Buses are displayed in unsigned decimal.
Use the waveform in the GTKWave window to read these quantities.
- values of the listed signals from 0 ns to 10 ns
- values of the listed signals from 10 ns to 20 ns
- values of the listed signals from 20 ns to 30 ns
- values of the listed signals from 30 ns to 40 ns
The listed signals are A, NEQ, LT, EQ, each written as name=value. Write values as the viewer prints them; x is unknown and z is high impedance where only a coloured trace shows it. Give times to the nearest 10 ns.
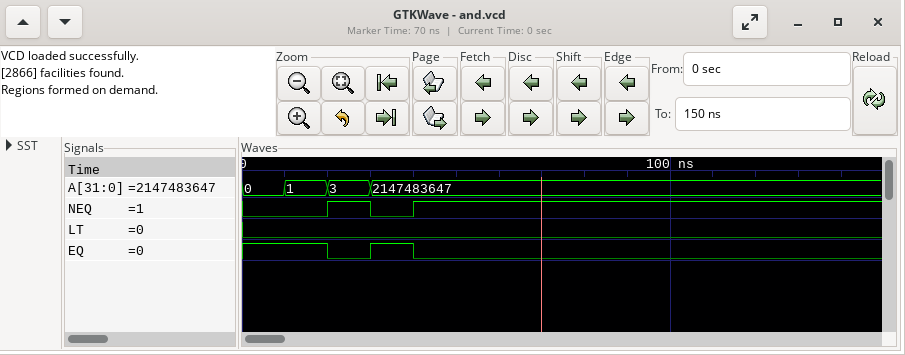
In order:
A=0, NEQ=0, LT=0, EQ=1
A=1, NEQ=0, LT=0, EQ=1
A=3, NEQ=1, LT=0, EQ=0
A=2147483647, NEQ=0, LT=0, EQ=1
